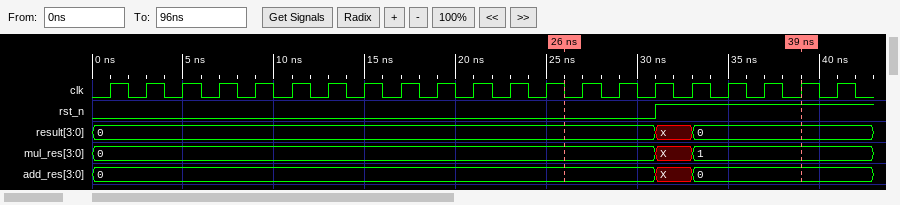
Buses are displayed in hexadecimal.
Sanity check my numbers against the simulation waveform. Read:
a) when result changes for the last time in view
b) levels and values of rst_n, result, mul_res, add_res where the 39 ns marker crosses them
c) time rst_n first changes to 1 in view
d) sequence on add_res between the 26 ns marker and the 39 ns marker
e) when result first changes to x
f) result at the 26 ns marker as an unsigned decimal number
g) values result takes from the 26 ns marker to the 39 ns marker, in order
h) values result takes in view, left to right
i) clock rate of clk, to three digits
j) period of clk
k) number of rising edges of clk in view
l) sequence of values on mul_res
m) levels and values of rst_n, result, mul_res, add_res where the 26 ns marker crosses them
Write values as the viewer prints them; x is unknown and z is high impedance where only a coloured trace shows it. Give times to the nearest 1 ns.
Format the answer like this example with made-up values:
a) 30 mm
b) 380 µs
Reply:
a) 33 ns
b) rst_n=1, result=0, mul_res=1, add_res=0
c) 31 ns
d) 0, X, 0
e) 31 ns
f) 0
g) 0, x, 0
h) 0, x, 0
i) 500 MHz
j) 2 ns
k) 21
l) 0, X, 1
m) rst_n=0, result=0, mul_res=0, add_res=0
